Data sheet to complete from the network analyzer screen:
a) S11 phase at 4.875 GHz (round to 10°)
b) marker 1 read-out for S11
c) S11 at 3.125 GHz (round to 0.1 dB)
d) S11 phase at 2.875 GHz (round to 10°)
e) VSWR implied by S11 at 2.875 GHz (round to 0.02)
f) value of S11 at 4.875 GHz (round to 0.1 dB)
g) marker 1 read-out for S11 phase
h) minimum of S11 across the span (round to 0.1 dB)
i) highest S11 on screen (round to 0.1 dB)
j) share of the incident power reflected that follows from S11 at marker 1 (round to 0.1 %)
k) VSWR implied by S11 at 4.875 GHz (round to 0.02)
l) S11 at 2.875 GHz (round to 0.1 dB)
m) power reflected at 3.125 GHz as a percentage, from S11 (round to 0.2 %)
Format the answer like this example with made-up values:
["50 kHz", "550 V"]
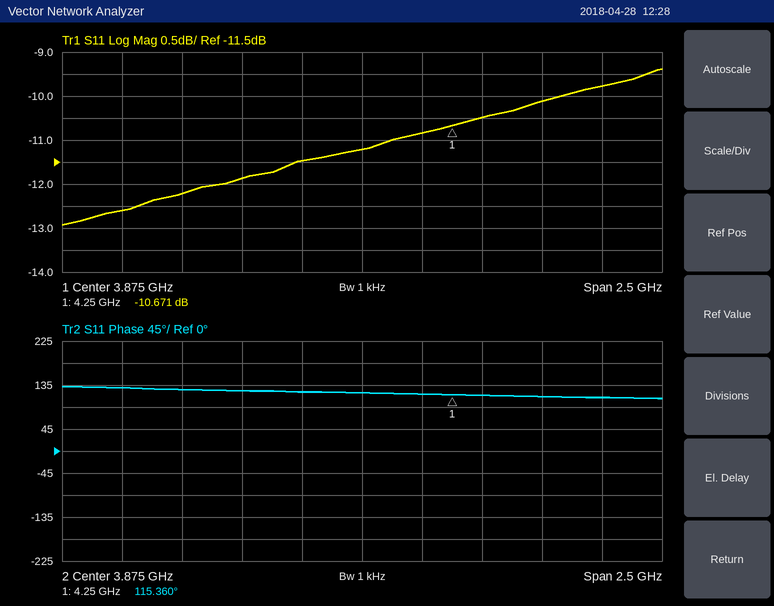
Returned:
["110°", "-10.671 dB", "-12.2 dB", "130°", "1.62", "-9.8 dB", "115.360°", "-12.9 dB", "-9.4 dB", "8.6 %", "1.96", "-12.6 dB", "6.0 %"]
